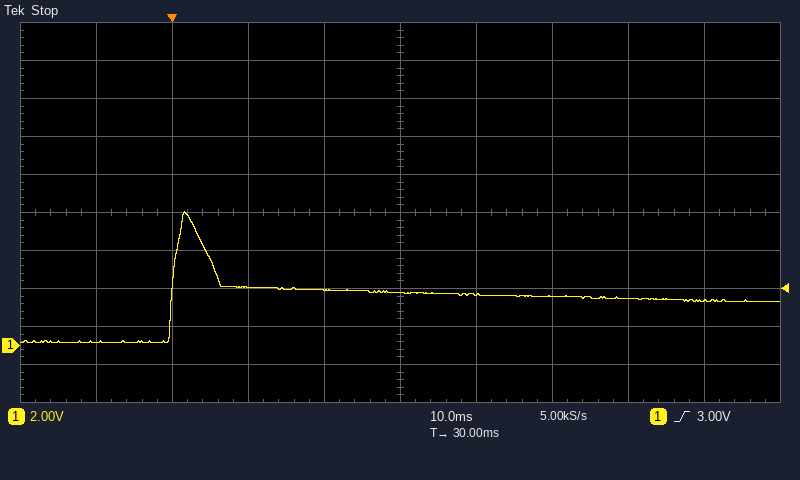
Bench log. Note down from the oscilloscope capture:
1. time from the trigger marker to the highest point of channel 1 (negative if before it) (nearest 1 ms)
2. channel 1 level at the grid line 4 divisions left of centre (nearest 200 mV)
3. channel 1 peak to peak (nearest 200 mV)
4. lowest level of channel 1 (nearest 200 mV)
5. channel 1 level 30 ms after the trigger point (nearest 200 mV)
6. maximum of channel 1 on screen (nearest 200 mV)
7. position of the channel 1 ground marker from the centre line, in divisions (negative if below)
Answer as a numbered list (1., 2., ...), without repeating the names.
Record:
1. +2 ms
2. 200 mV
3. 6.8 V
4. 200 mV
5. 2.8 V
6. 7.0 V
7. -3.5 div
